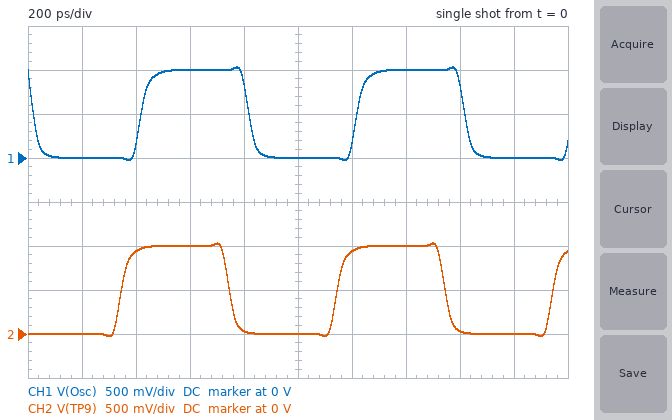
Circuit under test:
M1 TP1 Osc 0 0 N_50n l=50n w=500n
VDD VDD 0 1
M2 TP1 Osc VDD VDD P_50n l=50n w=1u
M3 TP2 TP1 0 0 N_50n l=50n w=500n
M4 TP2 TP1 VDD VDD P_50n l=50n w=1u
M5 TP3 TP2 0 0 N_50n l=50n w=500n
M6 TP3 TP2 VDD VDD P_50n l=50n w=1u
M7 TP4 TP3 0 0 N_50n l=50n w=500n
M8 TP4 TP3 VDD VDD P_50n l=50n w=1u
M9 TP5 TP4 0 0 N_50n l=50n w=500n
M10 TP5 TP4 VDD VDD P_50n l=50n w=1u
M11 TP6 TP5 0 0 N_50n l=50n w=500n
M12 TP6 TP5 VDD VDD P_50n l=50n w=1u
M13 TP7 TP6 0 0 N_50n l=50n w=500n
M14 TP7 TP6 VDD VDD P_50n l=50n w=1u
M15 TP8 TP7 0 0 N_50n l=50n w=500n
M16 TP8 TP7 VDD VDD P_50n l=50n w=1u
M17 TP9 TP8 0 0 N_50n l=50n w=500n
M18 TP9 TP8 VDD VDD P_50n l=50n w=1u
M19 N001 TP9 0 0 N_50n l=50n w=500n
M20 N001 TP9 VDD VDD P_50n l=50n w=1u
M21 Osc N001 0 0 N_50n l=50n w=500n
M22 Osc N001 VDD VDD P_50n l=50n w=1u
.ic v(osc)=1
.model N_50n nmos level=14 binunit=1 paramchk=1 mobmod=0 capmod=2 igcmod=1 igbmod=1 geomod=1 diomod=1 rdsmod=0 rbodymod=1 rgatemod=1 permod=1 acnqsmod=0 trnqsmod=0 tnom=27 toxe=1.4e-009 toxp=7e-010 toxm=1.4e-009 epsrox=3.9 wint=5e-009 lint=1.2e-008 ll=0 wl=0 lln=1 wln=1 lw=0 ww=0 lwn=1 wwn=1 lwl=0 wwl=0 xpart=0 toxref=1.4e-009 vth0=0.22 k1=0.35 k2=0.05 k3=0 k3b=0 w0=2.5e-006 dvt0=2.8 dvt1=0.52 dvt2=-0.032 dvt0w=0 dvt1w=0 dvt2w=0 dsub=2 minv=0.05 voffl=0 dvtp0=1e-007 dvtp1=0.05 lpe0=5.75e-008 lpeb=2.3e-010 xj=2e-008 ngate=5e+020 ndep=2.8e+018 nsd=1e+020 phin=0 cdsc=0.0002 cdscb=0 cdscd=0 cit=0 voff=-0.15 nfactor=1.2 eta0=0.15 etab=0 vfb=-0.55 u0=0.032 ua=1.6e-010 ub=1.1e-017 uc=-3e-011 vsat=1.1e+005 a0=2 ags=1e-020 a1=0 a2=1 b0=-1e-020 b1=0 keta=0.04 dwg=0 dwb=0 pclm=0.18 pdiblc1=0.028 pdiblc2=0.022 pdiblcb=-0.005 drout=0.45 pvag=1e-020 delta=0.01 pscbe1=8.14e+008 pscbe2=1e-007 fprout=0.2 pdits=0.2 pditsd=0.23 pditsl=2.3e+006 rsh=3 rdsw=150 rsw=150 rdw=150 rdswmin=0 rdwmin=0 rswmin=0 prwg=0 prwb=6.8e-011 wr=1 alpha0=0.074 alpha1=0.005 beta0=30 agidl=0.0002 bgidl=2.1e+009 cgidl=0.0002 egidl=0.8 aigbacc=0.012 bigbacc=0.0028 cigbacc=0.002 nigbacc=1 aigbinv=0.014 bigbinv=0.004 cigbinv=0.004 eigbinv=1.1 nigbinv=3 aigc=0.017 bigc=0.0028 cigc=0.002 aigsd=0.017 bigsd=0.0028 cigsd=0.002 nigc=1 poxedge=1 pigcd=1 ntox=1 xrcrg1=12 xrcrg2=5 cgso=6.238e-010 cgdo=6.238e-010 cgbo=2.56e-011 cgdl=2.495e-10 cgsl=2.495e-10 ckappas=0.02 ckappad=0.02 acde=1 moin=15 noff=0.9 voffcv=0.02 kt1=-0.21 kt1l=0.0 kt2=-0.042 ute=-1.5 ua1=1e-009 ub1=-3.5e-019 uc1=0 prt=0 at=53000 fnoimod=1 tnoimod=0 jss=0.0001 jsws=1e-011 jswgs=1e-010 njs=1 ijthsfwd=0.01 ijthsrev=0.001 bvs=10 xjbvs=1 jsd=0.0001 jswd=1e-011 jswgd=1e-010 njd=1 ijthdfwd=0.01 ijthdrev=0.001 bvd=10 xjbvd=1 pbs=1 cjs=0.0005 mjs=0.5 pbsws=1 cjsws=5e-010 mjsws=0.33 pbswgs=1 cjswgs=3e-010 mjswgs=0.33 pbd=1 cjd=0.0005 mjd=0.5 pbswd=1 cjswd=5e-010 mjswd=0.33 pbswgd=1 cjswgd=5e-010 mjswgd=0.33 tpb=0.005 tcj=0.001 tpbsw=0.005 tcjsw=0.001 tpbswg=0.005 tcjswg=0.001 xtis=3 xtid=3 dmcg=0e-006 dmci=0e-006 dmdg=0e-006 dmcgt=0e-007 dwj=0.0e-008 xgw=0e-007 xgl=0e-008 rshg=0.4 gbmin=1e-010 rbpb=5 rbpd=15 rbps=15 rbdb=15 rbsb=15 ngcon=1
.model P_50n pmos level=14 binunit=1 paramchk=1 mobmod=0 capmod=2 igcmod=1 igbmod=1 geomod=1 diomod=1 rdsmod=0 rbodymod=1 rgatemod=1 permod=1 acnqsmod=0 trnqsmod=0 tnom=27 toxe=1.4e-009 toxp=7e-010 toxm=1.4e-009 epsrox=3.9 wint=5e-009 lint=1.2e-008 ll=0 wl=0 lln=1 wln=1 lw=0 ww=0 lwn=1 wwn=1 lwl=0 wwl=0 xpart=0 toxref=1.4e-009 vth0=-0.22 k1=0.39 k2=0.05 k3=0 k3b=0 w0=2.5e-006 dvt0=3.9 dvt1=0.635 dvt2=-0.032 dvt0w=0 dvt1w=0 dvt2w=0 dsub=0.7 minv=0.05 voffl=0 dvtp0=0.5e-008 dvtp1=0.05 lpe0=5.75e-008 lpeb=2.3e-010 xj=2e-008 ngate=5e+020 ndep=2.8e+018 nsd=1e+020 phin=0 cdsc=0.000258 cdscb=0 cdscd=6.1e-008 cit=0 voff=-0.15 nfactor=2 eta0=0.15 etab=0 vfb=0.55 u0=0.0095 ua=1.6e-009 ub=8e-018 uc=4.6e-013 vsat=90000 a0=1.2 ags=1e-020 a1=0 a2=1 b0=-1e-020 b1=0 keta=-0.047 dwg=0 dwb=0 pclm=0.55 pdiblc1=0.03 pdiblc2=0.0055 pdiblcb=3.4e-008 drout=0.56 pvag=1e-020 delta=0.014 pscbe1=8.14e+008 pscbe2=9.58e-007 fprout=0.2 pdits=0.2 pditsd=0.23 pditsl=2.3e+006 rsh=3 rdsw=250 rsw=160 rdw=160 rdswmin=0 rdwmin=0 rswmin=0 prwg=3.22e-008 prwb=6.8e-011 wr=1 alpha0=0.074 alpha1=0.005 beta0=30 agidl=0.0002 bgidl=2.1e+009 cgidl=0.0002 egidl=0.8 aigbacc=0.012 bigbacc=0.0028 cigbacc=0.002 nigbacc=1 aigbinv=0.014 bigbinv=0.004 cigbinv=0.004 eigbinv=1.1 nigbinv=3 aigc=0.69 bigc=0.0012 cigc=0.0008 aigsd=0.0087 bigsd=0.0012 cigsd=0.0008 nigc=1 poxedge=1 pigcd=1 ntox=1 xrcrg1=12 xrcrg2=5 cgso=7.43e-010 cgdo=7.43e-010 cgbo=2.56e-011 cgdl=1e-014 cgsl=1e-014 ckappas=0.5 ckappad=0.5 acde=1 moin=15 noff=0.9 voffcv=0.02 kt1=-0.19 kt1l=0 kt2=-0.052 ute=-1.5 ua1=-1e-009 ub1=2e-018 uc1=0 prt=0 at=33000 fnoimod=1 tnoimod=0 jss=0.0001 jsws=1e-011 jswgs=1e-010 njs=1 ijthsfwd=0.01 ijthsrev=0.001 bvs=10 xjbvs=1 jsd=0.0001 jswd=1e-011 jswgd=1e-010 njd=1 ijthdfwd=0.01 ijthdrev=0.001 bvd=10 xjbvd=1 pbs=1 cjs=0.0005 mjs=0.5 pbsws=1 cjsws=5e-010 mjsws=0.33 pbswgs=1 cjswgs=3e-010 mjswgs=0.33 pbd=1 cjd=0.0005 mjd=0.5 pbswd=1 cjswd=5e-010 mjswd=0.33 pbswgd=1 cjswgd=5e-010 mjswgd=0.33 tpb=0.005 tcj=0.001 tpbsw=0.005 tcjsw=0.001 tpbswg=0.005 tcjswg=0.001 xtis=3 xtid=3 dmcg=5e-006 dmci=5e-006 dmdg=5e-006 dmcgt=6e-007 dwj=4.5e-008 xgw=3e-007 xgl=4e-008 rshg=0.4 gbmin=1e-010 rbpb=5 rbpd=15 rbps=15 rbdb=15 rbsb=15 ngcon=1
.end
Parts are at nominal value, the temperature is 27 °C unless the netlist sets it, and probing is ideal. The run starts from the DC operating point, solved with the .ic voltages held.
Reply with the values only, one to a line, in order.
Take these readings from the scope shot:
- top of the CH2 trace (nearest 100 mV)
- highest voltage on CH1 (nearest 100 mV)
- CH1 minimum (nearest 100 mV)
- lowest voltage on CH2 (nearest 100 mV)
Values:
1.0 V
1.0 V
0 V
0 V
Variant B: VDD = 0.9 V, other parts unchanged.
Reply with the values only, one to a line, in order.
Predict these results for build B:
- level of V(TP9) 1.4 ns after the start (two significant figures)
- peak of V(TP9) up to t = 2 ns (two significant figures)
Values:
890 mV
930 mV
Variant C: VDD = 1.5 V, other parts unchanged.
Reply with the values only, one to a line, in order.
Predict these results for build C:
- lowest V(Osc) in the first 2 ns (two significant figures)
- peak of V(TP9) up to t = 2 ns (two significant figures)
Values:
-26 mV
1.5 V
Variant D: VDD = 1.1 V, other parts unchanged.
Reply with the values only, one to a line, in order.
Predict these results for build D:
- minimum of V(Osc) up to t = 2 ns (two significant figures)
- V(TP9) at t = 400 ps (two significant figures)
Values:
-24 mV
1.1 V
